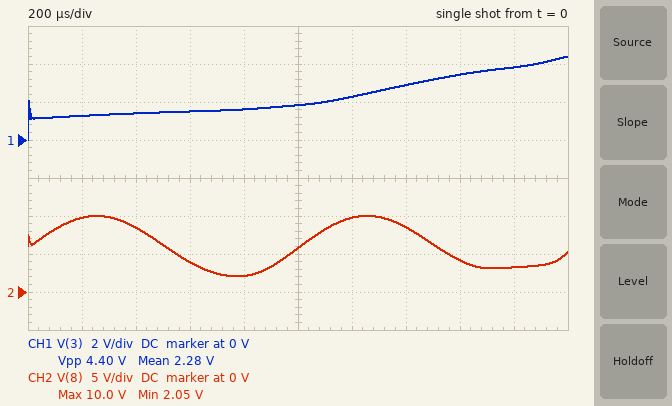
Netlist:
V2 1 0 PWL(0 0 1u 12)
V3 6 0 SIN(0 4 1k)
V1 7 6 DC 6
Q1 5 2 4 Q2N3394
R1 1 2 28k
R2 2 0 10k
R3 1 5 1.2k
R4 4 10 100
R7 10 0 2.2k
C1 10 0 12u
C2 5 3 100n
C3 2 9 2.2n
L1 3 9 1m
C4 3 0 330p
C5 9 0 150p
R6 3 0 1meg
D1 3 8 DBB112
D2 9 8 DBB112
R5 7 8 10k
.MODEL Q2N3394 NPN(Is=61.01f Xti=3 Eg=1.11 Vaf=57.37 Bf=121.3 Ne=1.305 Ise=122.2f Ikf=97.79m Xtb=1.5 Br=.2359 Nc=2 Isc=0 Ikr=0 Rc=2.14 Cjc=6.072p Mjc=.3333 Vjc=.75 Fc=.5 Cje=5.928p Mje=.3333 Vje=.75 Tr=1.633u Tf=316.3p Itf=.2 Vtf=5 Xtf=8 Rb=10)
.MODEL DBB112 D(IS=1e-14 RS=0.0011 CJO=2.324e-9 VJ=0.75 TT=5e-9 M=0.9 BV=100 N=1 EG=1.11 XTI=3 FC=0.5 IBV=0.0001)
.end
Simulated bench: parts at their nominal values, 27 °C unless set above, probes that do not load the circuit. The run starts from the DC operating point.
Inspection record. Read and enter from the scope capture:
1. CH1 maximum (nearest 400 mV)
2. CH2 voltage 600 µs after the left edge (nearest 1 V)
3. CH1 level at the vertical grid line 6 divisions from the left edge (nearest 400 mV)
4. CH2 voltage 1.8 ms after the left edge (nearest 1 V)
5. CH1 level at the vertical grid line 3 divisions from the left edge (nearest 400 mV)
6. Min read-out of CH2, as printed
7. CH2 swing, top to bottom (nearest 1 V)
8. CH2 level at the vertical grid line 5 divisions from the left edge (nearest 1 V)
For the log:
4.4 V
4 V
2.4 V
3 V
1.6 V
2.05 V
8 V
6 V
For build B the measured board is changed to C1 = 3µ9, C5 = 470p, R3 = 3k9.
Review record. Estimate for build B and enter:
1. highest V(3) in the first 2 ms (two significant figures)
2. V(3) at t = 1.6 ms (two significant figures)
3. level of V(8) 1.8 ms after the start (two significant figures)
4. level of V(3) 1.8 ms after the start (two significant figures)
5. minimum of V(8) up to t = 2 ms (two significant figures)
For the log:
1.7 V
1.5 V
2.1 V
1.6 V
2.0 V
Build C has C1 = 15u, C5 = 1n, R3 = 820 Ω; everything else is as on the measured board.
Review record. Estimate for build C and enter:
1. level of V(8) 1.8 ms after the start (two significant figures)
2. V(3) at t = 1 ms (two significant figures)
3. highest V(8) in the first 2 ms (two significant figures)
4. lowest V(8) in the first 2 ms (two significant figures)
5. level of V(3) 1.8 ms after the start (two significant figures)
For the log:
4.6 V
4.2 V
11 V
3.0 V
5.2 V
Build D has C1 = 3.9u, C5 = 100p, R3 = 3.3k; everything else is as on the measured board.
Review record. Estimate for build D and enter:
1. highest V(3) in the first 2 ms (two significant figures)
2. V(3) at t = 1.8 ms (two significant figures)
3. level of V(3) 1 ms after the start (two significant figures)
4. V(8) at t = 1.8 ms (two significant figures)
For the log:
2.0 V
1.8 V
1.3 V
2.1 V
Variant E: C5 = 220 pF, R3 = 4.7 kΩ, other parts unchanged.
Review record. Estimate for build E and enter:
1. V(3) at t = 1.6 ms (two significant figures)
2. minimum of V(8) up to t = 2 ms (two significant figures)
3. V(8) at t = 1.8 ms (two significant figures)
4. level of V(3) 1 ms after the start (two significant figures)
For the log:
700 mV
2.0 V
2.1 V
600 mV
